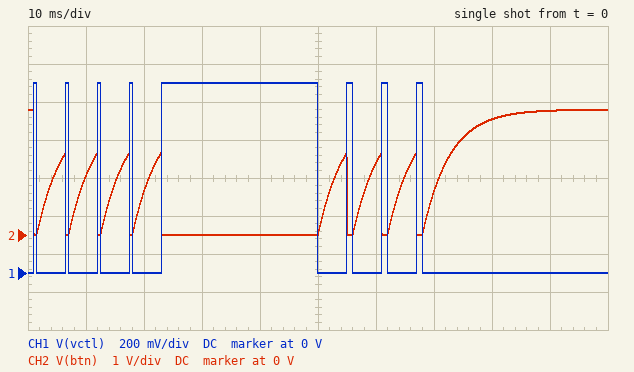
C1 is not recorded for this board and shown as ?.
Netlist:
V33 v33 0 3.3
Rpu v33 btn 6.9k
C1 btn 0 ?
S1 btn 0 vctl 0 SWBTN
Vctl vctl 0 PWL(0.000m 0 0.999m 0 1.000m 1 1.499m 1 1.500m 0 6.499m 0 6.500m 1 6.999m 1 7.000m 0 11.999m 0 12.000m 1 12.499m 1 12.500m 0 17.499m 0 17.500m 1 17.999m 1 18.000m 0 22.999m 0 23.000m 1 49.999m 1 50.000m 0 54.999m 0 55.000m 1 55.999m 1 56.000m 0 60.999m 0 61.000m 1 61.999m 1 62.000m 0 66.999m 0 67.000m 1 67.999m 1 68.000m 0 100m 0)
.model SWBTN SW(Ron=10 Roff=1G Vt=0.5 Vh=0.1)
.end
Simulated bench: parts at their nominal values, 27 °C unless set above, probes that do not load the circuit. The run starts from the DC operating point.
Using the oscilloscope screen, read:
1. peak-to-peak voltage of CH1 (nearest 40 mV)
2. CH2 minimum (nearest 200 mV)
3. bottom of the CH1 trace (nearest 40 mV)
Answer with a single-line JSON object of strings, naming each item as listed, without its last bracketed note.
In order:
{"peak-to-peak voltage of CH1": "1.00 V", "CH2 minimum": "0 V", "bottom of the CH1 trace": "0 V"}
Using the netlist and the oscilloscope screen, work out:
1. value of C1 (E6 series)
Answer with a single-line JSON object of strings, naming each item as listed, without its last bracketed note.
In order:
{"value of C1": "680 nF"}
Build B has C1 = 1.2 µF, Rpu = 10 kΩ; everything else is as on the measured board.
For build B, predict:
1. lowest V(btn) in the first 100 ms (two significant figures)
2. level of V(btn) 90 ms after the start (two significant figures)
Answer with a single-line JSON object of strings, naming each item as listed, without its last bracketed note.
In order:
{"lowest V(btn) in the first 100 ms": "3.3 mV", "level of V(btn) 90 ms after the start": "2.8 V"}
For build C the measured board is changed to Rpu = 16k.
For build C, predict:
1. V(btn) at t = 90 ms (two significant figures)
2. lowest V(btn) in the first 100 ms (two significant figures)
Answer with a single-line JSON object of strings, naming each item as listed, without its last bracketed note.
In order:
{"V(btn) at t = 90 ms": "2.9 V", "lowest V(btn) in the first 100 ms": "2.1 mV"}
